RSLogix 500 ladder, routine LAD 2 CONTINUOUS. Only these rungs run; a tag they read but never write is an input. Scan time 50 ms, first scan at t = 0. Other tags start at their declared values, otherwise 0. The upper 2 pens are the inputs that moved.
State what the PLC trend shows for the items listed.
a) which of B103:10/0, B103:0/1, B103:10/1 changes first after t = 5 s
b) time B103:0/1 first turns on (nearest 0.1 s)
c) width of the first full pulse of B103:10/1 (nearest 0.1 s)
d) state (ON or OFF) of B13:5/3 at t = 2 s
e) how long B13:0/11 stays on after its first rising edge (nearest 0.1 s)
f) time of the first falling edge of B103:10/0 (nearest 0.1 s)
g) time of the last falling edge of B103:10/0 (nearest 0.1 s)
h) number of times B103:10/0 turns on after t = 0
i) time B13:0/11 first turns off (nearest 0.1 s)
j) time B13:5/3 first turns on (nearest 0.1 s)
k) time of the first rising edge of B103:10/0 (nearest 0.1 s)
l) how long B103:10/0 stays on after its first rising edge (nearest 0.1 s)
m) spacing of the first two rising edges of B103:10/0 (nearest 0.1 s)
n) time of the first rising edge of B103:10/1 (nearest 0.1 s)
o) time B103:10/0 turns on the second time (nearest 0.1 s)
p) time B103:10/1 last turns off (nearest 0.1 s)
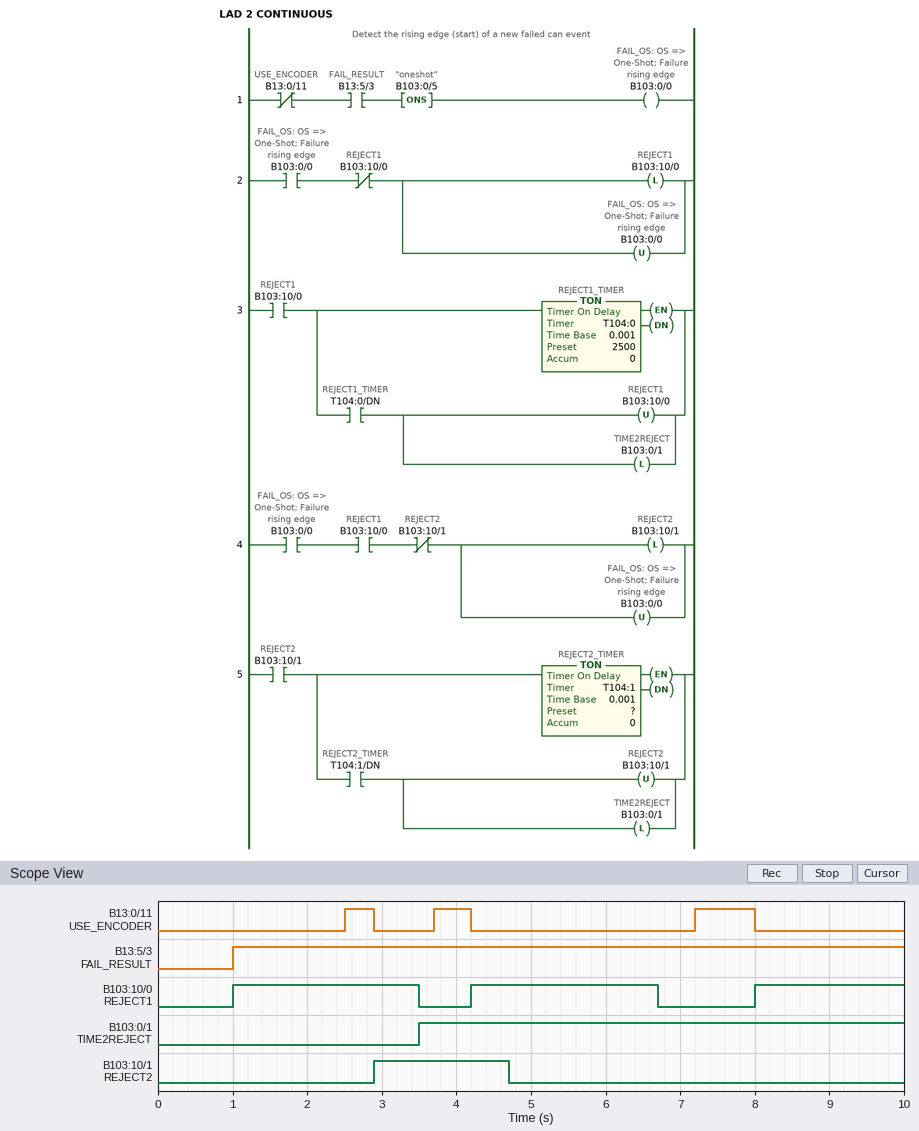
B103:10/0
3.5 s
1.8 s
ON
0.4 s
3.5 s
6.7 s
3
2.9 s
1.0 s
1.0 s
2.5 s
3.2 s
2.9 s
4.2 s
4.7 s
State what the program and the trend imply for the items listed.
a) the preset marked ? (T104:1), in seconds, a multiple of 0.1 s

1.8 s
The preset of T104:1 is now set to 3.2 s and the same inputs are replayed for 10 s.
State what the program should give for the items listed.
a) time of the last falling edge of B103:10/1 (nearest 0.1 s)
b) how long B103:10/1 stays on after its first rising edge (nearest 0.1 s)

6.1 s
3.2 s
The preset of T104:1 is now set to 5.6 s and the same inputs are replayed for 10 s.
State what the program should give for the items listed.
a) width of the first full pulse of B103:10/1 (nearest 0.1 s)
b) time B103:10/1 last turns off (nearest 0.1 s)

5.6 s
8.5 s
